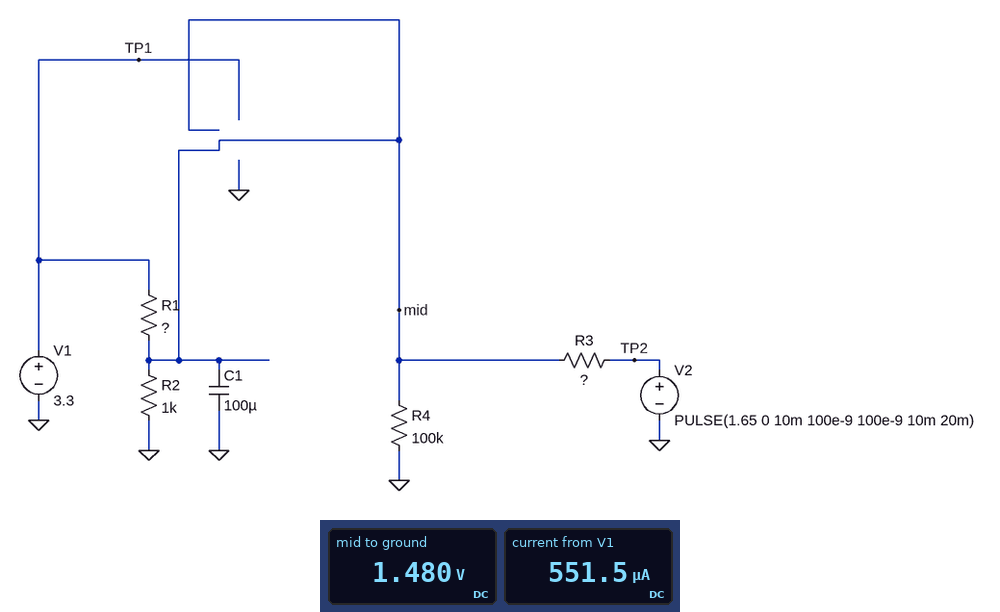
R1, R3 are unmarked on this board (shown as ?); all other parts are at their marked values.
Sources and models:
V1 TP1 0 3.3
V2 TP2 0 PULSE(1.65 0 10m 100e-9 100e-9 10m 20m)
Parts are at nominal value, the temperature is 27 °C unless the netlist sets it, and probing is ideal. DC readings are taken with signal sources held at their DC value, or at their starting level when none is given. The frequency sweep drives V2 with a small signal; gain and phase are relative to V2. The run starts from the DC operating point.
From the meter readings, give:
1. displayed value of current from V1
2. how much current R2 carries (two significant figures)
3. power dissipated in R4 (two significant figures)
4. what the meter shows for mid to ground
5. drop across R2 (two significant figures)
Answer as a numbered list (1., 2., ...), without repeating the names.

1. 551.5 µA
2. 1.5 mA
3. 22 µW
4. 1.480 V
5. 1.5 V
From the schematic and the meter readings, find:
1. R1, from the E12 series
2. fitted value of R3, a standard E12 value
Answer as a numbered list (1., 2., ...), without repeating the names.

1. 3.3 kΩ
2. 180 Ω
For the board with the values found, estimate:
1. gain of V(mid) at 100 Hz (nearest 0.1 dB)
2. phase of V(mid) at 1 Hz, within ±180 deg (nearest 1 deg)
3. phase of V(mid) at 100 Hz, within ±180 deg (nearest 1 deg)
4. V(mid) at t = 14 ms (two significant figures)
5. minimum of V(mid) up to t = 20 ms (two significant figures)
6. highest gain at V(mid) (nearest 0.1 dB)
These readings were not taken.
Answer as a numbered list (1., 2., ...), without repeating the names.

1. -21.1 dB
2. -5 deg
3. -84 deg
4. 1.2 V
5. 820 mV
6. -1.8 dB
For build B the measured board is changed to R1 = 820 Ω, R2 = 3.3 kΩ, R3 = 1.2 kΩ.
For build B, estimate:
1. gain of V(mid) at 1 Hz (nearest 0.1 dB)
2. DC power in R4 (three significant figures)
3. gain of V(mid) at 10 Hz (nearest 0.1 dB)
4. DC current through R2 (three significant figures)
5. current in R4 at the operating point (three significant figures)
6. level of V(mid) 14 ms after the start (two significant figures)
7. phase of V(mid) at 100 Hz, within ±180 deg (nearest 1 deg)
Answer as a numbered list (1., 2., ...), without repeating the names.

1. -9.4 dB
2. 52.1 µW
3. -18.1 dB
4. 692 µA
5. 22.8 µA
6. 2.2 V
7. -88 deg
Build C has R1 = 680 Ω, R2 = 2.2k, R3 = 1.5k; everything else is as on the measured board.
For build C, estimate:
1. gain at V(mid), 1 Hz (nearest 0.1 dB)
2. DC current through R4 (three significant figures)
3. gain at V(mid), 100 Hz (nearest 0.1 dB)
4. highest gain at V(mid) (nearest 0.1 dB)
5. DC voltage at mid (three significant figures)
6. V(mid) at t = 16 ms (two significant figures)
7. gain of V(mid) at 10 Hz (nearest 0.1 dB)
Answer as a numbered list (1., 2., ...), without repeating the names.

1. -12.1 dB
2. 22.9 µA
3. -39.5 dB
4. -11.8 dB
5. 2.29 V
6. 2.2 V
7. -20.2 dB
